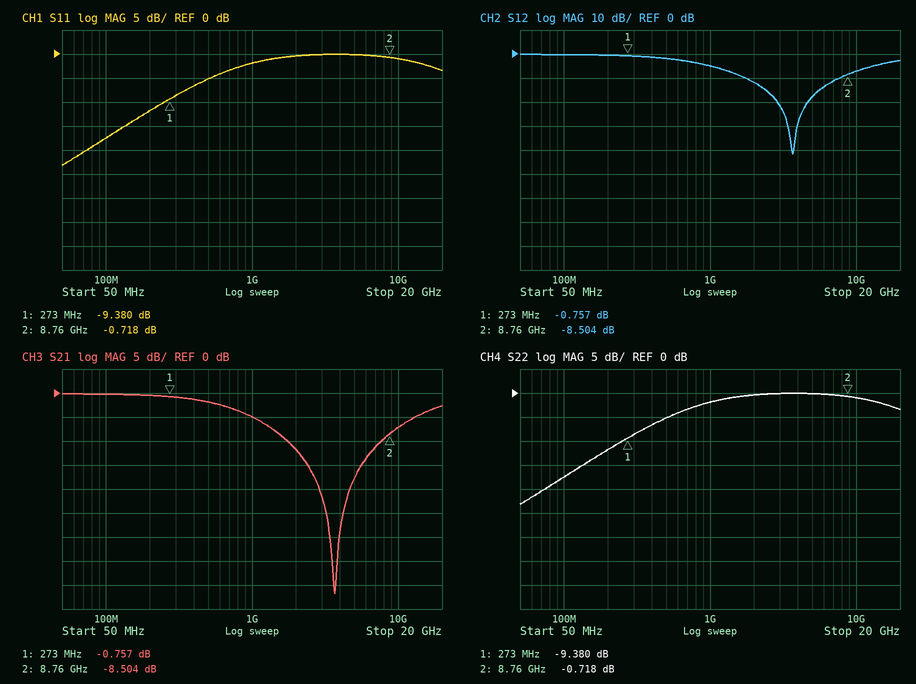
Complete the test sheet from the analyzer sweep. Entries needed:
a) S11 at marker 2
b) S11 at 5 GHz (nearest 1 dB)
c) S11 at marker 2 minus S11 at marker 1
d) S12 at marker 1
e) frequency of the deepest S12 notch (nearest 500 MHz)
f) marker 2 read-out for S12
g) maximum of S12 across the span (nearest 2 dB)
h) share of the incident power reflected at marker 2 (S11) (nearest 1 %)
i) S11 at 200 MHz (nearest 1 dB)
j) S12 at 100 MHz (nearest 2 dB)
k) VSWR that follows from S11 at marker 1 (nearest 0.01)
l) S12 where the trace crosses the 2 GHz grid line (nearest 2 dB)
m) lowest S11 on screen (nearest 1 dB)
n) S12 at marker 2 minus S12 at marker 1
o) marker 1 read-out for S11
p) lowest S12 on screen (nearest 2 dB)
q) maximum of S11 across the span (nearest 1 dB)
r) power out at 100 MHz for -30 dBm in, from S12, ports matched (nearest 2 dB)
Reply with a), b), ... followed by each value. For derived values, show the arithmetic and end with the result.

a) -0.718 dB
b) 0 dB
c) -0.718 − (-9.38) = 8.662 dB
d) -0.757 dB
e) 3.5 GHz
f) -8.504 dB
g) 0 dB
h) 10^(-0.718/10) ≈ 85 %
i) -12 dB
j) 0 dB
k) (1 + 0.3396)/(1 − 0.3396) ≈ 2.03
l) -12 dB
m) -23 dB
n) -8.504 − (-0.757) = -7.747 dB
o) -9.380 dB
p) -42 dB
q) 0 dB
r) -30 dBm + (0 dB) = -30 dBm
